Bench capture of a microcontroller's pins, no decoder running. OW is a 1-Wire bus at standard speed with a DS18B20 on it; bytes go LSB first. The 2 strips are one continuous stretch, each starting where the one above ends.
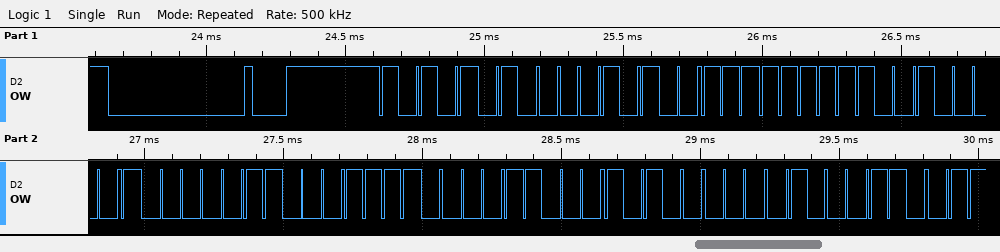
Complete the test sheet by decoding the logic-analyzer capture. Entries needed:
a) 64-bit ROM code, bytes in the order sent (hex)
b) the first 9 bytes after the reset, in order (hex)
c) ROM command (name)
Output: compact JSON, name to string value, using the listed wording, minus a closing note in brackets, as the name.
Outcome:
{"64-bit ROM code, bytes in the order sent": "28 FF 09 C1 78 18 05 62", "the first 9 bytes after the reset, in order": "55 28 FF 09 C1 78 18 05 62", "ROM command": "Match ROM"}
